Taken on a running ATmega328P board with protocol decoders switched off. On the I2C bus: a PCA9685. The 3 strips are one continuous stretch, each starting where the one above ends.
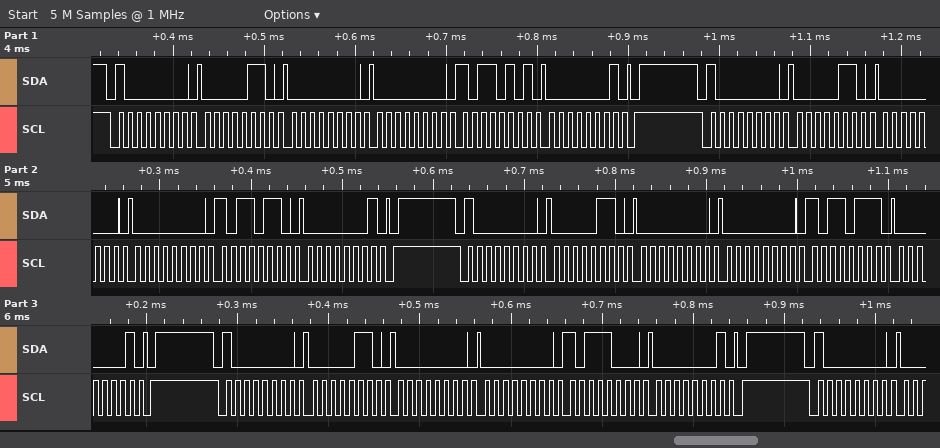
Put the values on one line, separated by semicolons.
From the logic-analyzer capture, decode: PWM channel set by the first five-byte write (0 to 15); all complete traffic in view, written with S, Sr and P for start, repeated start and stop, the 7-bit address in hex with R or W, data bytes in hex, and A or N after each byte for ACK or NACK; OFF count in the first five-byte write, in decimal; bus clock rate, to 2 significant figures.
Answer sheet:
0; S 40W A 06 A 00 A 00 A B5 A 01 A P S 40W A 06 A 00 A 00 A B6 A 01 A P S 40W A 06 A 00 A 00 A B7 A 01 A P S 40W A 06 A 00 A 00 A B8 A 01 A P S 40W A; 437; 100 kHz
